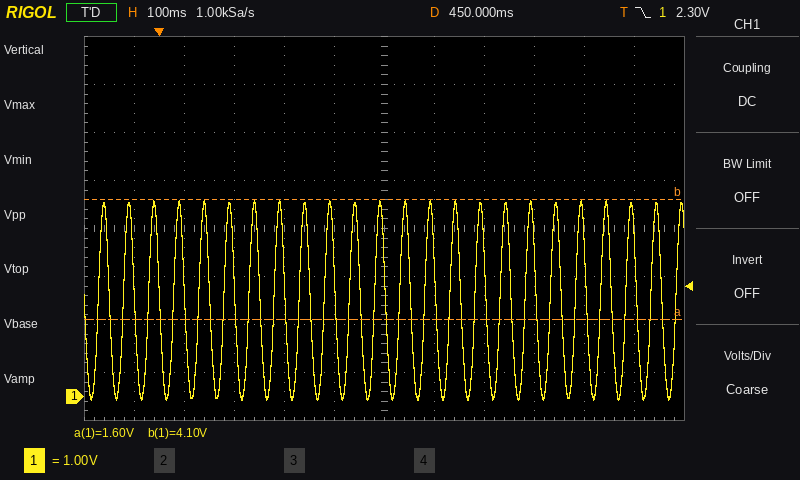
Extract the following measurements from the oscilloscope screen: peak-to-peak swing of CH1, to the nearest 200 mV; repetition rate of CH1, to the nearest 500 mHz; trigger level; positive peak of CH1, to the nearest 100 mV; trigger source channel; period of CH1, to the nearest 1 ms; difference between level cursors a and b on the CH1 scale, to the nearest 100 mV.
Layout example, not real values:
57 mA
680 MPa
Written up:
4.2 V
20.0 Hz
2.30 V
4.1 V
CH1
50 ms
2.5 V
